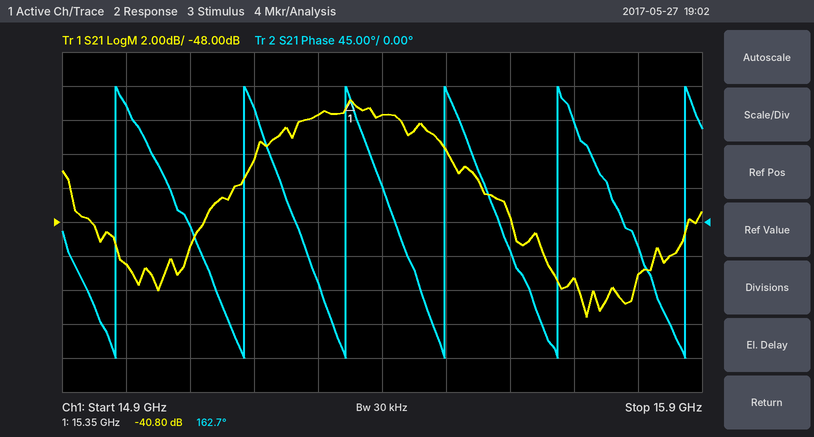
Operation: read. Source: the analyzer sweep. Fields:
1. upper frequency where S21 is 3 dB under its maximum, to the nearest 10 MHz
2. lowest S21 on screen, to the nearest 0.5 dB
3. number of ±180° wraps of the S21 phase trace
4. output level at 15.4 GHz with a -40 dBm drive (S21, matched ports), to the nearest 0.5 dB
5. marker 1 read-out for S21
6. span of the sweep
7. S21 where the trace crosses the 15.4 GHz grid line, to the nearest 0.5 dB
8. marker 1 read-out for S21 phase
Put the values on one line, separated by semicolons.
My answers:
15.50 GHz; -53.5 dB; 6; -81.5 dBm; -40.80 dB; 1 GHz; -41.5 dB; 162.7°
